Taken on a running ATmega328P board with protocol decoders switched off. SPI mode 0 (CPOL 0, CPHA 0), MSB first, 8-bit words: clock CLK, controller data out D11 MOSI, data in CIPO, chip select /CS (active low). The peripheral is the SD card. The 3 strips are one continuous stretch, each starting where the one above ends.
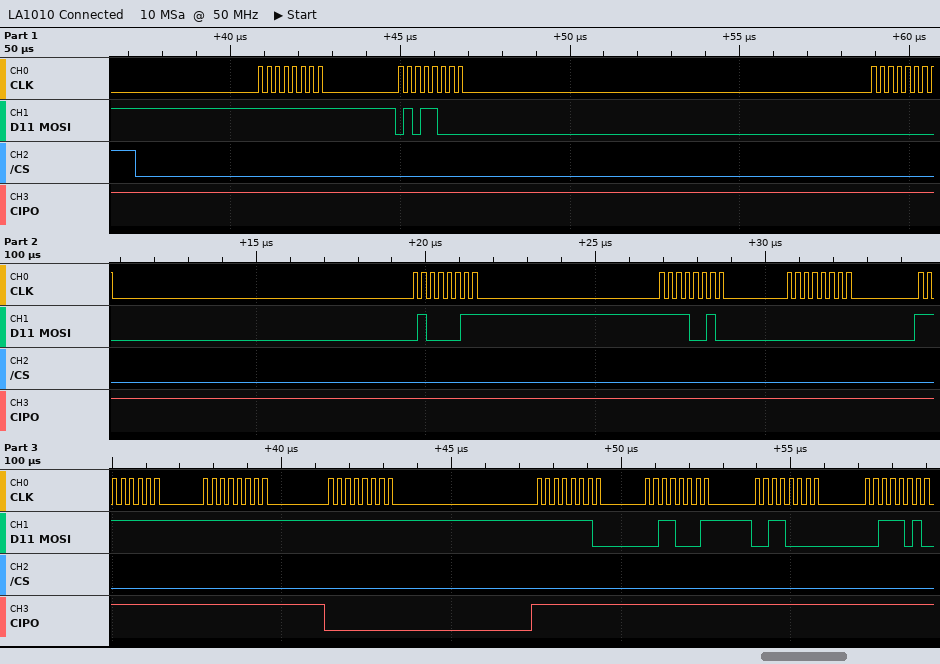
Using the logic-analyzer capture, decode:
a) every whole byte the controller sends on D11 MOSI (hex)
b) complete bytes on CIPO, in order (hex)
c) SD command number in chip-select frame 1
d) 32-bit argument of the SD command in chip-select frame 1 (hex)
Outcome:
0xFF 0x58 0x00 0x43 0xF2 0x00 0xFF 0xFF 0xFF 0xFE 0x31 0x30 0x3A
0xFF 0xFF 0xFF 0xFF 0xFF 0xFF 0xFF 0xFF 0x00 0xFF 0xFF 0xFF 0xFF
CMD24
0x0043F200
